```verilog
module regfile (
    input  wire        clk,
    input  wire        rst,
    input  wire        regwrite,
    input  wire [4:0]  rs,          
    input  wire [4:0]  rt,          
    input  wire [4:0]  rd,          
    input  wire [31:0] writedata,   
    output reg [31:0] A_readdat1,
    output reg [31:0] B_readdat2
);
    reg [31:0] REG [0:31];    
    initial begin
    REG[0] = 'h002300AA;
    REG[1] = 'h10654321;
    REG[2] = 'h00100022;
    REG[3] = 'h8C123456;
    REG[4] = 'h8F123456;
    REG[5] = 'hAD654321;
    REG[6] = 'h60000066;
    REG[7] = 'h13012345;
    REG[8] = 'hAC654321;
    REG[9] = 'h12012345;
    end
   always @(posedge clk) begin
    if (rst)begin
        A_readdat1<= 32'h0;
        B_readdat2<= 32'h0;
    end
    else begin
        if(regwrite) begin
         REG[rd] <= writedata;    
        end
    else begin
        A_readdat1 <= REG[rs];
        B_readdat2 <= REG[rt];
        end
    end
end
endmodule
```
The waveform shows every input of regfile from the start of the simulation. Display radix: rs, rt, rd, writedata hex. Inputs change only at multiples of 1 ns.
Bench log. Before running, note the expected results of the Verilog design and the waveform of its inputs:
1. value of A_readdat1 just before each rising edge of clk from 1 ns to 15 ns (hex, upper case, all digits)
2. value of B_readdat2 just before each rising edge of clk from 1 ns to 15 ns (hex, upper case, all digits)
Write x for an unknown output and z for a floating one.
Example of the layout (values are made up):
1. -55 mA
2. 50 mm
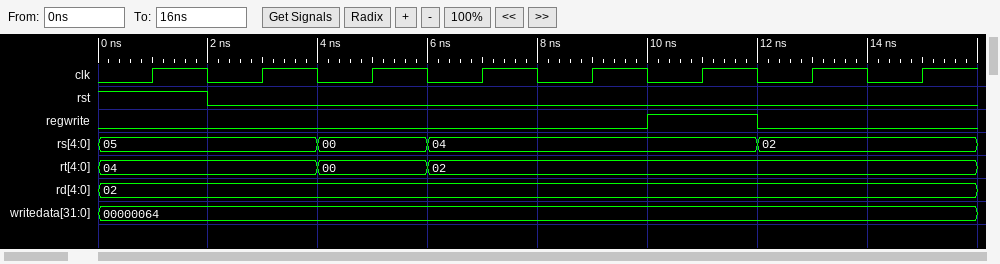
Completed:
1. x, 00000000, AD654321, 002300AA, 8F123456, 8F123456, 8F123456, 00000064
2. x, 00000000, 8F123456, 002300AA, 00100022, 00100022, 00100022, 00000064
